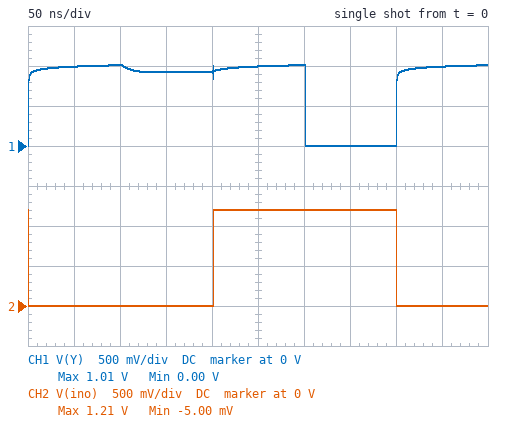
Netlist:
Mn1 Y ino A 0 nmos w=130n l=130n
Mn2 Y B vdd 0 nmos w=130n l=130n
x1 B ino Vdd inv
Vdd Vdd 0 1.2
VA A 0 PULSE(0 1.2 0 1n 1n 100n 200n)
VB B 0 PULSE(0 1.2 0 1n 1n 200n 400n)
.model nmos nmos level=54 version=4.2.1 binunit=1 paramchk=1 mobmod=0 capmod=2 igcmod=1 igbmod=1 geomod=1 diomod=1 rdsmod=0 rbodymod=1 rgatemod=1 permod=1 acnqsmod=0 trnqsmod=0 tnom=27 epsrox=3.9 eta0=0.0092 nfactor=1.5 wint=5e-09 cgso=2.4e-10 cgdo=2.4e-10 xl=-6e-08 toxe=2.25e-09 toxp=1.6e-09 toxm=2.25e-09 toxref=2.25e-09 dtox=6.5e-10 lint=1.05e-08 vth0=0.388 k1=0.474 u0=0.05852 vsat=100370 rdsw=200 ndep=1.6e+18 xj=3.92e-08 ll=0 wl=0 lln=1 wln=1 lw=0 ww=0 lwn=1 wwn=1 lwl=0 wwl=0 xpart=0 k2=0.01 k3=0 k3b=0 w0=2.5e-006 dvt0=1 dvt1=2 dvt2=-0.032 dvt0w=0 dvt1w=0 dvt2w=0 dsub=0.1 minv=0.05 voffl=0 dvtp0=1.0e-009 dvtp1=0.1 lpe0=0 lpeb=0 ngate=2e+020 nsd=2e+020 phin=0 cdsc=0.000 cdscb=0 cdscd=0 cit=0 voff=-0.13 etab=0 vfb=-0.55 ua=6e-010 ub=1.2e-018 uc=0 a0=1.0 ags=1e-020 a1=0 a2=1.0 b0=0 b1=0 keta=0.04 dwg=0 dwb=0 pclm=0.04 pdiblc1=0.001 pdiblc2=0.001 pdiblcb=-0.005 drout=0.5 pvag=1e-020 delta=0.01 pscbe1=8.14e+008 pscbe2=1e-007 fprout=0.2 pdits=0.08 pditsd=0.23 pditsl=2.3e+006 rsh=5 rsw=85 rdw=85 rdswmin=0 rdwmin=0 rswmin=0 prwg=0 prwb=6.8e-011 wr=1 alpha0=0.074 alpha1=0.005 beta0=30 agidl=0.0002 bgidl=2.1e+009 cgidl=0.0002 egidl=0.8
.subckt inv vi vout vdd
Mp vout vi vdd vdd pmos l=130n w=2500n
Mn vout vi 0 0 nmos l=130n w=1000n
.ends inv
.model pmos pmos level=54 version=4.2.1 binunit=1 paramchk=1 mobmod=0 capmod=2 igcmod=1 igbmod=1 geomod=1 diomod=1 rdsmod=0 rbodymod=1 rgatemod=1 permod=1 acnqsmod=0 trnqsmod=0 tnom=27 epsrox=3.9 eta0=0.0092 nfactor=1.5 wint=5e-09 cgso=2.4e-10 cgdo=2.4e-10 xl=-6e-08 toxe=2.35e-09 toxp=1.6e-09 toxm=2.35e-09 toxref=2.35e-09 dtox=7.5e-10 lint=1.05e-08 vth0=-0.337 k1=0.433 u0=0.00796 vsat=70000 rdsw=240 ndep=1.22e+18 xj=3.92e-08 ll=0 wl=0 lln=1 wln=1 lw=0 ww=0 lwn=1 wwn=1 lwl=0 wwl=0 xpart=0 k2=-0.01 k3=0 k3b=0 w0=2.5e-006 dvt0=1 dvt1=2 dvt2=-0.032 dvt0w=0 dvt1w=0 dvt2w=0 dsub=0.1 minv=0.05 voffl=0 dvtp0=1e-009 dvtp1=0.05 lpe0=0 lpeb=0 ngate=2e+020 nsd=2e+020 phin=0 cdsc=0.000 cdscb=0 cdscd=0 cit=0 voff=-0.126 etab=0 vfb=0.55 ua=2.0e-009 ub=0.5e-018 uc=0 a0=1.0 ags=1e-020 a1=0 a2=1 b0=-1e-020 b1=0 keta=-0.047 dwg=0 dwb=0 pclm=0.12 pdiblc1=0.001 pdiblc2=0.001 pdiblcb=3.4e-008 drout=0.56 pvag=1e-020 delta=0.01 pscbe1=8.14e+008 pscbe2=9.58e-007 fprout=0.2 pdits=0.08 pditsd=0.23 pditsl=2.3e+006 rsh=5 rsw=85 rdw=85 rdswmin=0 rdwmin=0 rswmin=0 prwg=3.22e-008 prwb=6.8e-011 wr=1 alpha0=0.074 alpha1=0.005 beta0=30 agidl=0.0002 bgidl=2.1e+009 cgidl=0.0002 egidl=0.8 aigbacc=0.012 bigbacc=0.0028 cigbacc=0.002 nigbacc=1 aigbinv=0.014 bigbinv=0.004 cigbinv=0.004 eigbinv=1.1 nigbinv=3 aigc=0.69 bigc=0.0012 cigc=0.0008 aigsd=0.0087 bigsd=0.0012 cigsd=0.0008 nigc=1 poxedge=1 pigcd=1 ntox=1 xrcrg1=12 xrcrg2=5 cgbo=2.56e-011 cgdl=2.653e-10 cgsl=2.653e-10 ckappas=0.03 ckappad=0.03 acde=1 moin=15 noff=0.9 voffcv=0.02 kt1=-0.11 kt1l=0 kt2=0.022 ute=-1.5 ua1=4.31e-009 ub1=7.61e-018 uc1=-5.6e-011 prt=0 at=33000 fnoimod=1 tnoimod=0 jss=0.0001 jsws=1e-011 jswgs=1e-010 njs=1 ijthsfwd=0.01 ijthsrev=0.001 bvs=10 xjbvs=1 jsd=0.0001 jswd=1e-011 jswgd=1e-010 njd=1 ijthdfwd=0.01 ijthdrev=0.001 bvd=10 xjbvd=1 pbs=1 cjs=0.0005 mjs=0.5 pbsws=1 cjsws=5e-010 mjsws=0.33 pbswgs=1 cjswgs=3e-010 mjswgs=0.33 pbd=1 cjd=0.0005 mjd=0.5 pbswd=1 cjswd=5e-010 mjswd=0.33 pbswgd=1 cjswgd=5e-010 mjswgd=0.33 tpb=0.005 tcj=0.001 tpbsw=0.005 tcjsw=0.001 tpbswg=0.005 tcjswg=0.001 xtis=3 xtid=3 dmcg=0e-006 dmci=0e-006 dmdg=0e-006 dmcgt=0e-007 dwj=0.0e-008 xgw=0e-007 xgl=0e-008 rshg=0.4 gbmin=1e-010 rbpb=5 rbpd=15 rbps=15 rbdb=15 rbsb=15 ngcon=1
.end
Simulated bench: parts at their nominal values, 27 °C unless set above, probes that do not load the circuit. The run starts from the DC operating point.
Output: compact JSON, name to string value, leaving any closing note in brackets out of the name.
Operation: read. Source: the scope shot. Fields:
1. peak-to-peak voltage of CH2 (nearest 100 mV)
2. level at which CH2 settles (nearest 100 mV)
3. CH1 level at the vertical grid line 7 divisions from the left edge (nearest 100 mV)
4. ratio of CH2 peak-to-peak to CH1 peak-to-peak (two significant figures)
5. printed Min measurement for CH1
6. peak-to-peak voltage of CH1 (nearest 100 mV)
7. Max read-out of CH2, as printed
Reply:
{"peak-to-peak voltage of CH2": "1.2 V", "level at which CH2 settles": "0 V", "CH1 level at the vertical grid line 7 divisions from the left edge": "0 V", "ratio of CH2 peak-to-peak to CH1 peak-to-peak": "1.2", "printed Min measurement for CH1": "0.00 V", "peak-to-peak voltage of CH1": "1.0 V", "Max read-out of CH2, as printed": "1.21 V"}
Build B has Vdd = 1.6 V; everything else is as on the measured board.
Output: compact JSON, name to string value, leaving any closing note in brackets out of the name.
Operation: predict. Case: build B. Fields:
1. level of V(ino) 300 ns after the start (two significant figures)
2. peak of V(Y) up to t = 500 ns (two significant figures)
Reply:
{"level of V(ino) 300 ns after the start": "1.6 V", "peak of V(Y) up to t = 500 ns": "1.2 V"}
